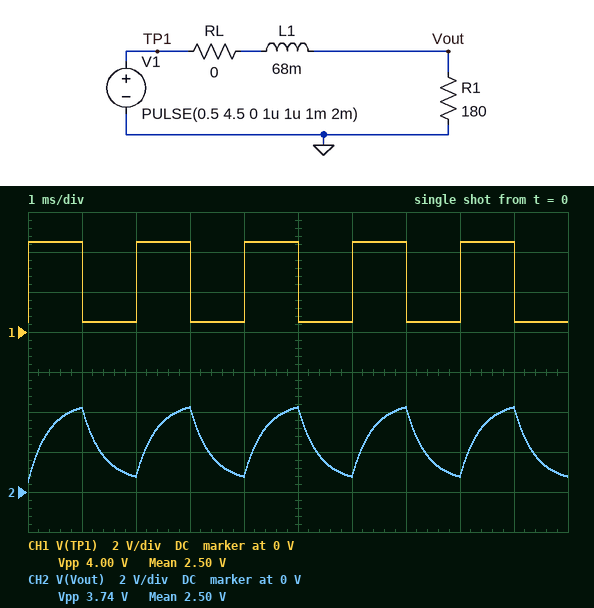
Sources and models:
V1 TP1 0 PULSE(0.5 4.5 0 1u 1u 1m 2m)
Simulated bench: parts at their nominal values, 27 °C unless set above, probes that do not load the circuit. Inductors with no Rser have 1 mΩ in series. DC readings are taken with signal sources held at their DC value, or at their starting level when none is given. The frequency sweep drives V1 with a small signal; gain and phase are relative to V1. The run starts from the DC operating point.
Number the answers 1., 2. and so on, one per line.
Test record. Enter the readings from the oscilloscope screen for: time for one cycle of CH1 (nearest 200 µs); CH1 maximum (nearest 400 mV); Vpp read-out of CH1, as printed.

1. 2.0 ms
2. 4.4 V
3. 4.00 V
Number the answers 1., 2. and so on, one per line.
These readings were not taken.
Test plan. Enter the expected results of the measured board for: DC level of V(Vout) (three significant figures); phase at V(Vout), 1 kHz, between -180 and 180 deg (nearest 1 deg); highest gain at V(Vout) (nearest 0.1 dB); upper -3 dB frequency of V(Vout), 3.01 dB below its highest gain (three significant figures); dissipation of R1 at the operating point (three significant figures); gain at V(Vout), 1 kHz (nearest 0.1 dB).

1. 500 mV
2. -67 deg
3. 0 dB
4. 421 Hz
5. 1.39 mW
6. -8.2 dB
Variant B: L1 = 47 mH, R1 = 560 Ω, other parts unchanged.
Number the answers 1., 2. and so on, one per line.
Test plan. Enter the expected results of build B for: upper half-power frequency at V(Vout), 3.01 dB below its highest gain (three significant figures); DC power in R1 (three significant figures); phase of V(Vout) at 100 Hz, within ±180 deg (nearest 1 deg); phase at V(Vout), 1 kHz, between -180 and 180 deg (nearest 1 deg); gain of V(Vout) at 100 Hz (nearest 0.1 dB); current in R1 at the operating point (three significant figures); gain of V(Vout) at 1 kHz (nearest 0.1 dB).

1. 1.90 kHz
2. 446 µW
3. -3 deg
4. -28 deg
5. 0 dB
6. 893 µA
7. -1.1 dB
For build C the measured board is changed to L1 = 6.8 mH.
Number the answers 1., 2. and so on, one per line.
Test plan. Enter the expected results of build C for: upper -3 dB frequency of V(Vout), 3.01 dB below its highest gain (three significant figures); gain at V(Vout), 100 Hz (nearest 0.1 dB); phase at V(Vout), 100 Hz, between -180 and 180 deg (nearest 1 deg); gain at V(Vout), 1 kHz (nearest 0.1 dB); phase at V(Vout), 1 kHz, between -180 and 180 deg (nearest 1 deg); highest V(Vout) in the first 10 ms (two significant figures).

1. 4.21 kHz
2. 0 dB
3. -1 deg
4. -0.2 dB
5. -13 deg
6. 4.5 V
